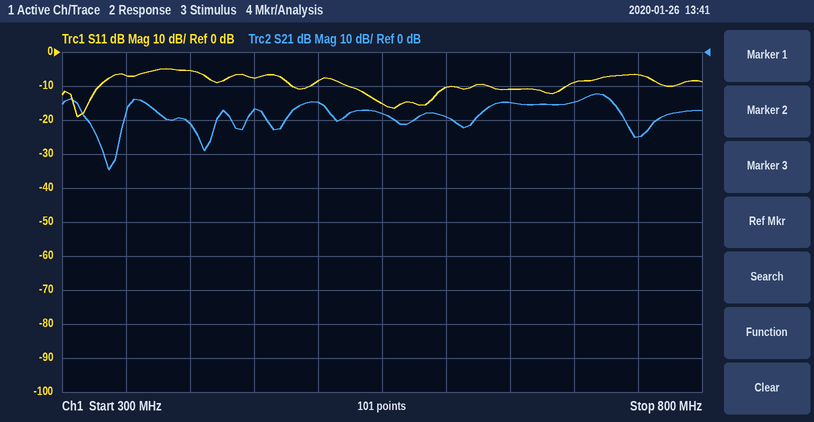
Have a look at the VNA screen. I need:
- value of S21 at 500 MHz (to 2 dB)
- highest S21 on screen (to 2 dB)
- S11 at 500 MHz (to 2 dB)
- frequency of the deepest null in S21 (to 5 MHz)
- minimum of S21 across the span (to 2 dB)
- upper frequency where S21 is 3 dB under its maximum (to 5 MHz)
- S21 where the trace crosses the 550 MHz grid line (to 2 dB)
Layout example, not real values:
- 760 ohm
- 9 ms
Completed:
- -14 dB
- -12 dB
- -8 dB
- 335 MHz
- -34 dB
- 730 MHz
- -18 dB
